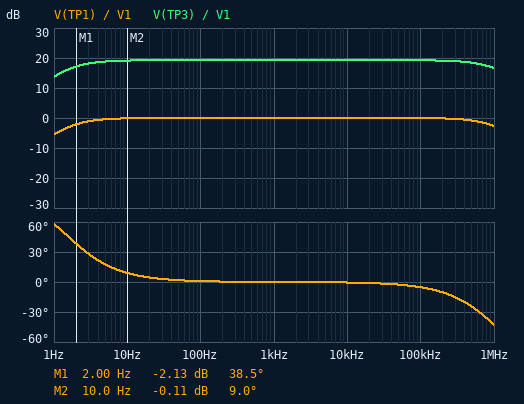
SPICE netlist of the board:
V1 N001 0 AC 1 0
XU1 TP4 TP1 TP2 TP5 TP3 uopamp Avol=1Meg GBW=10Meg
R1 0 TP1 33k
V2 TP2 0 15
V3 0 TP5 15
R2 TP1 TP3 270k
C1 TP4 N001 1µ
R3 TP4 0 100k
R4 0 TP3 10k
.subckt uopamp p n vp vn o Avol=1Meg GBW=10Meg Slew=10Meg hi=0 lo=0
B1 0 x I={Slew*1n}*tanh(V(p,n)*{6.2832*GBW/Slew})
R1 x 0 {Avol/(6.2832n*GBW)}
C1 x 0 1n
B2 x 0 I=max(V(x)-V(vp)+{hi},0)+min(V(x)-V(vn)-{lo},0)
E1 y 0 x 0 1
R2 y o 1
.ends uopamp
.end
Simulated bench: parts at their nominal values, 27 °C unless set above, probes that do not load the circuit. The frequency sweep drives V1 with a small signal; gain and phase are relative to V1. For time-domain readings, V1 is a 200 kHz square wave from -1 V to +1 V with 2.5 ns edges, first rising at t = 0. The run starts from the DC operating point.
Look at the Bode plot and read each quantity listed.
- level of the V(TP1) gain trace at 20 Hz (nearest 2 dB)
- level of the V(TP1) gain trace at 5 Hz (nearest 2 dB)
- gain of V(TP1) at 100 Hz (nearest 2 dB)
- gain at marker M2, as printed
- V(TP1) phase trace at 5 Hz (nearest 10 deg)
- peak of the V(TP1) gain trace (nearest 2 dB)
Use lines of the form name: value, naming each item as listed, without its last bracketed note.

level of the V(TP1) gain trace at 20 Hz: 0 dB
level of the V(TP1) gain trace at 5 Hz: 0 dB
gain of V(TP1) at 100 Hz: 0 dB
gain at marker M2, as printed: -0.11 dB
V(TP1) phase trace at 5 Hz: 20 deg
peak of the V(TP1) gain trace: 0 dB
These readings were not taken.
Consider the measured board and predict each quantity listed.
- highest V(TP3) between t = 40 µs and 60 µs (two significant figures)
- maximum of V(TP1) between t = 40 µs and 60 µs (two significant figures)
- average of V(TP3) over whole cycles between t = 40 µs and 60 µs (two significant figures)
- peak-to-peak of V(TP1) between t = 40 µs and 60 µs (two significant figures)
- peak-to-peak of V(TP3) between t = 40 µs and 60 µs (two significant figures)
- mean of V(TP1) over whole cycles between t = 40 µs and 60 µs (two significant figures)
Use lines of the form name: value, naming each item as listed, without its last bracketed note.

highest V(TP3) between t = 40 µs and 60 µs: 15 V
maximum of V(TP1) between t = 40 µs and 60 µs: 1.6 V
average of V(TP3) over whole cycles between t = 40 µs and 60 µs: 7.5 V
peak-to-peak of V(TP1) between t = 40 µs and 60 µs: 1.6 V
peak-to-peak of V(TP3) between t = 40 µs and 60 µs: 15 V
mean of V(TP1) over whole cycles between t = 40 µs and 60 µs: 820 mV
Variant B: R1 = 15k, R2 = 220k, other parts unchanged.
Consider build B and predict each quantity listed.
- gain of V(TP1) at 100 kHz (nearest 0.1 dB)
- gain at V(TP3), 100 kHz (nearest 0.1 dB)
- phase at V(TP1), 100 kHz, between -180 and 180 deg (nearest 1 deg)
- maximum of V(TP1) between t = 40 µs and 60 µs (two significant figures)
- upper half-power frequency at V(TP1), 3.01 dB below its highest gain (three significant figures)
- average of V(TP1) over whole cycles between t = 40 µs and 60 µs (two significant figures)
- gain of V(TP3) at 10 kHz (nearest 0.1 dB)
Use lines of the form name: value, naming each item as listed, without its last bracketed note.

gain of V(TP1) at 100 kHz: -0.1 dB
gain at V(TP3), 100 kHz: 23.8 dB
phase at V(TP1), 100 kHz, between -180 and 180 deg: -9 deg
maximum of V(TP1) between t = 40 µs and 60 µs: 960 mV
upper half-power frequency at V(TP1), 3.01 dB below its highest gain: 638 kHz
average of V(TP1) over whole cycles between t = 40 µs and 60 µs: 490 mV
gain of V(TP3) at 10 kHz: 23.9 dB
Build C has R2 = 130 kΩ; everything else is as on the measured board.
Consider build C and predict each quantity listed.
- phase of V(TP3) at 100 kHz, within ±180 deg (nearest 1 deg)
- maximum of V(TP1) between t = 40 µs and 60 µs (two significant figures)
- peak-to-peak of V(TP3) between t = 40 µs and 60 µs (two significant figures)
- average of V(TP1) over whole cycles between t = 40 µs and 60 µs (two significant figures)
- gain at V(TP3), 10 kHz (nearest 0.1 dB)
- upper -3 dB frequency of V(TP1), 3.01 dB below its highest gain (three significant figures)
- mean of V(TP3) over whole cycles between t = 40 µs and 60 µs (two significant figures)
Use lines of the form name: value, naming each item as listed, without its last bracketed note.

phase of V(TP3) at 100 kHz, within ±180 deg: -3 deg
maximum of V(TP1) between t = 40 µs and 60 µs: 2.0 V
peak-to-peak of V(TP3) between t = 40 µs and 60 µs: 9.9 V
average of V(TP1) over whole cycles between t = 40 µs and 60 µs: 1.0 V
gain at V(TP3), 10 kHz: 13.9 dB
upper -3 dB frequency of V(TP1), 3.01 dB below its highest gain: 2.02 MHz
mean of V(TP3) over whole cycles between t = 40 µs and 60 µs: 4.9 V
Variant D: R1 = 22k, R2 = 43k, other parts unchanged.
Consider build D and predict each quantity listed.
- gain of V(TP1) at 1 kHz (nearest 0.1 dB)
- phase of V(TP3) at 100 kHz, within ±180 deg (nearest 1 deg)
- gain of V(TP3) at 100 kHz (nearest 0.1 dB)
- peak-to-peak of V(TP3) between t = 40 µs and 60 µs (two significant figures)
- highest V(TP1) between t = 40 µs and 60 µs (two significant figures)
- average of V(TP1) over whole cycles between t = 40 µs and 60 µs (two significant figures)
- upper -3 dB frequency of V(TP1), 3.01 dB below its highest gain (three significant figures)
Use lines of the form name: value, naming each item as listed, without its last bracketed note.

gain of V(TP1) at 1 kHz: 0 dB
phase of V(TP3) at 100 kHz, within ±180 deg: -2 deg
gain of V(TP3) at 100 kHz: 9.4 dB
peak-to-peak of V(TP3) between t = 40 µs and 60 µs: 5.9 V
highest V(TP1) between t = 40 µs and 60 µs: 2.0 V
average of V(TP1) over whole cycles between t = 40 µs and 60 µs: 1.0 V
upper -3 dB frequency of V(TP1), 3.01 dB below its highest gain: 3.38 MHz
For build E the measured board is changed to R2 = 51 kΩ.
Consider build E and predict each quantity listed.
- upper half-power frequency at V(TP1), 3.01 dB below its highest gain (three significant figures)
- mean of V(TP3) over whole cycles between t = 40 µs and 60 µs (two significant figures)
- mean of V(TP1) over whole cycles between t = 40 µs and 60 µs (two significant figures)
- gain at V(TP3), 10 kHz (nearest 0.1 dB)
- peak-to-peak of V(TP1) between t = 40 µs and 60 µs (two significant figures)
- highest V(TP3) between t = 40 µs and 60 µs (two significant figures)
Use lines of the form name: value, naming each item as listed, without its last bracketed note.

upper half-power frequency at V(TP1), 3.01 dB below its highest gain: 3.93 MHz
mean of V(TP3) over whole cycles between t = 40 µs and 60 µs: 2.5 V
mean of V(TP1) over whole cycles between t = 40 µs and 60 µs: 1.0 V
gain at V(TP3), 10 kHz: 8.1 dB
peak-to-peak of V(TP1) between t = 40 µs and 60 µs: 2.0 V
highest V(TP3) between t = 40 µs and 60 µs: 5.1 V
